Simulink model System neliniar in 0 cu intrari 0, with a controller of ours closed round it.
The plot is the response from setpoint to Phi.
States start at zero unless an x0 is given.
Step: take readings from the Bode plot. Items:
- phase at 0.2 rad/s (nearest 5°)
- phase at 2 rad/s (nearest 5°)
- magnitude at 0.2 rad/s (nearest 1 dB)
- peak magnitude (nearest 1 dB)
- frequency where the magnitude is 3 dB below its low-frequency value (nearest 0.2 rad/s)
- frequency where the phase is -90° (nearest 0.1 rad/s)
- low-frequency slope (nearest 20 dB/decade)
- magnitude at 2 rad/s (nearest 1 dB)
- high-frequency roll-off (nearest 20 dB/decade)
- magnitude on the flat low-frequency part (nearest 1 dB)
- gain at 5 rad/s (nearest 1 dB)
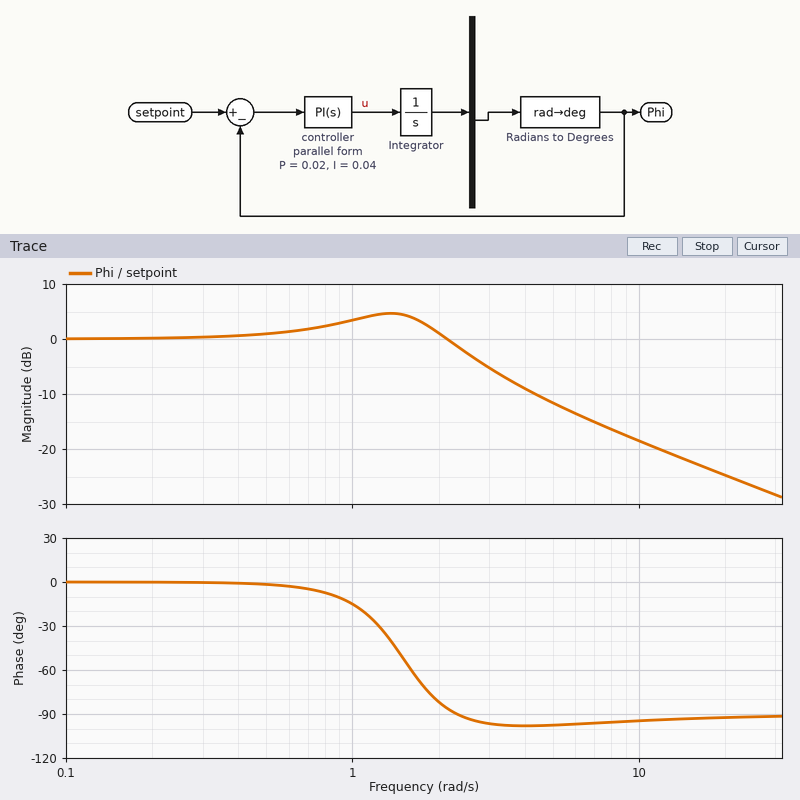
0°
-80°
0 dB
5 dB
2.6 rad/s
2.3 rad/s
0 dB/decade
1 dB
-20 dB/decade
0 dB
-12 dB
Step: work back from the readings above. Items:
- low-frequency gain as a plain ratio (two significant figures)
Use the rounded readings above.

1.0
